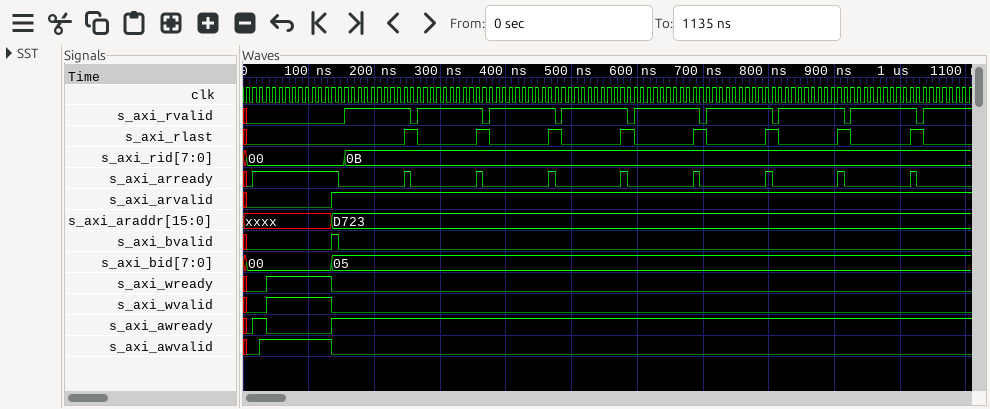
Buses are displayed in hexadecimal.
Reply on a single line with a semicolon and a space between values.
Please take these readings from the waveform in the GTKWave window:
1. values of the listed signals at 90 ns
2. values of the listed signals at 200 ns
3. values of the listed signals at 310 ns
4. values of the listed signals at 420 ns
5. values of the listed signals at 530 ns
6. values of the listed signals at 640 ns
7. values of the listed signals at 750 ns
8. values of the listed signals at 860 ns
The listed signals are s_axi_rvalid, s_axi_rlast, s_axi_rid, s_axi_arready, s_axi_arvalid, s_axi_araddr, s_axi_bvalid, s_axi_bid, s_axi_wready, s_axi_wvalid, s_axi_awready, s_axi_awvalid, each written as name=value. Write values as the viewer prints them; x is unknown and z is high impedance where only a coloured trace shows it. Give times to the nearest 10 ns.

s_axi_rvalid=0, s_axi_rlast=0, s_axi_rid=00, s_axi_arready=1, s_axi_arvalid=0, s_axi_araddr=xxxx, s_axi_bvalid=0, s_axi_bid=00, s_axi_wready=1, s_axi_wvalid=1, s_axi_awready=0, s_axi_awvalid=1; s_axi_rvalid=1, s_axi_rlast=0, s_axi_rid=0B, s_axi_arready=0, s_axi_arvalid=1, s_axi_araddr=D723, s_axi_bvalid=0, s_axi_bid=05, s_axi_wready=0, s_axi_wvalid=0, s_axi_awready=1, s_axi_awvalid=0; s_axi_rvalid=1, s_axi_rlast=0, s_axi_rid=0B, s_axi_arready=0, s_axi_arvalid=1, s_axi_araddr=D723, s_axi_bvalid=0, s_axi_bid=05, s_axi_wready=0, s_axi_wvalid=0, s_axi_awready=1, s_axi_awvalid=0; s_axi_rvalid=1, s_axi_rlast=0, s_axi_rid=0B, s_axi_arready=0, s_axi_arvalid=1, s_axi_araddr=D723, s_axi_bvalid=0, s_axi_bid=05, s_axi_wready=0, s_axi_wvalid=0, s_axi_awready=1, s_axi_awvalid=0; s_axi_rvalid=1, s_axi_rlast=0, s_axi_rid=0B, s_axi_arready=0, s_axi_arvalid=1, s_axi_araddr=D723, s_axi_bvalid=0, s_axi_bid=05, s_axi_wready=0, s_axi_wvalid=0, s_axi_awready=1, s_axi_awvalid=0; s_axi_rvalid=1, s_axi_rlast=0, s_axi_rid=0B, s_axi_arready=0, s_axi_arvalid=1, s_axi_araddr=D723, s_axi_bvalid=0, s_axi_bid=05, s_axi_wready=0, s_axi_wvalid=0, s_axi_awready=1, s_axi_awvalid=0; s_axi_rvalid=1, s_axi_rlast=0, s_axi_rid=0B, s_axi_arready=0, s_axi_arvalid=1, s_axi_araddr=D723, s_axi_bvalid=0, s_axi_bid=05, s_axi_wready=0, s_axi_wvalid=0, s_axi_awready=1, s_axi_awvalid=0; s_axi_rvalid=1, s_axi_rlast=0, s_axi_rid=0B, s_axi_arready=0, s_axi_arvalid=1, s_axi_araddr=D723, s_axi_bvalid=0, s_axi_bid=05, s_axi_wready=0, s_axi_wvalid=0, s_axi_awready=1, s_axi_awvalid=0
